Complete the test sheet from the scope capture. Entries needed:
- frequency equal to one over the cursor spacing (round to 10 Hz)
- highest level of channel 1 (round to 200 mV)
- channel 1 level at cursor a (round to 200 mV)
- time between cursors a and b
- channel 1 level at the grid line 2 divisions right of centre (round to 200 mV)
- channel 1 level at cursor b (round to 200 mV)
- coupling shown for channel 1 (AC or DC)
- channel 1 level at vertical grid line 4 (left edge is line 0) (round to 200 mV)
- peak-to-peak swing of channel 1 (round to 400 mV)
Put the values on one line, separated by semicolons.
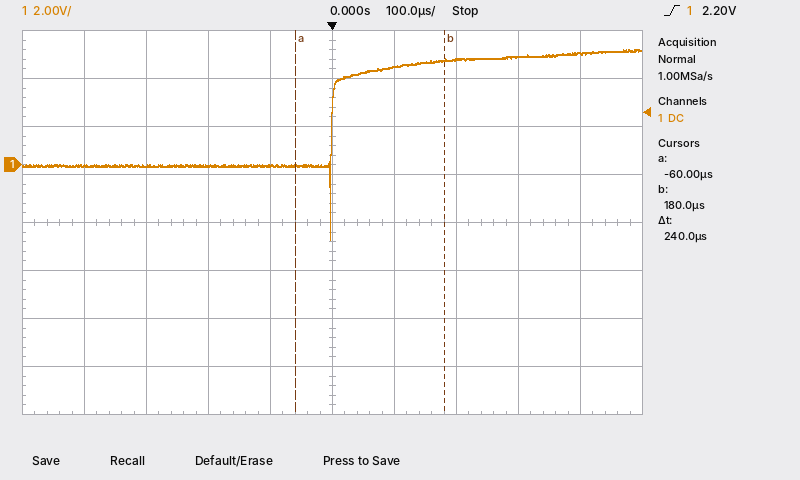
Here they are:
4.17 kHz; 4.8 V; 0.0 V; 240 µs; 4.4 V; 4.4 V; DC; 0.0 V; 8.0 V
